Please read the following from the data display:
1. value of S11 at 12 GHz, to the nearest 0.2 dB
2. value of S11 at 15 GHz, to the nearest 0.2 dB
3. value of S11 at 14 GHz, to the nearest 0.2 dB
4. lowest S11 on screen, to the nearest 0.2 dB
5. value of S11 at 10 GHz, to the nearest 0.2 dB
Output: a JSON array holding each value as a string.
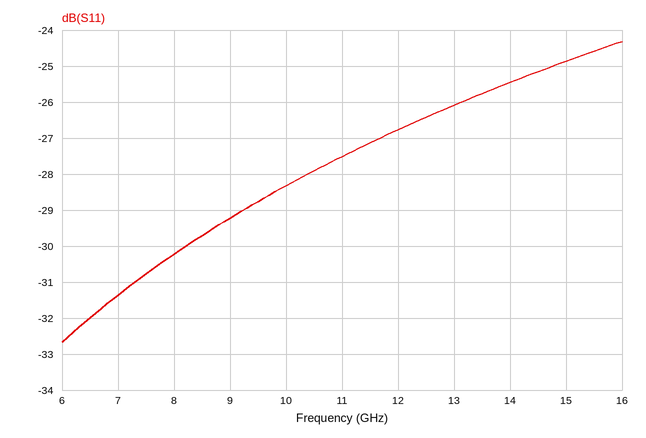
["-26.8 dB", "-24.8 dB", "-25.4 dB", "-32.6 dB", "-28.4 dB"]
